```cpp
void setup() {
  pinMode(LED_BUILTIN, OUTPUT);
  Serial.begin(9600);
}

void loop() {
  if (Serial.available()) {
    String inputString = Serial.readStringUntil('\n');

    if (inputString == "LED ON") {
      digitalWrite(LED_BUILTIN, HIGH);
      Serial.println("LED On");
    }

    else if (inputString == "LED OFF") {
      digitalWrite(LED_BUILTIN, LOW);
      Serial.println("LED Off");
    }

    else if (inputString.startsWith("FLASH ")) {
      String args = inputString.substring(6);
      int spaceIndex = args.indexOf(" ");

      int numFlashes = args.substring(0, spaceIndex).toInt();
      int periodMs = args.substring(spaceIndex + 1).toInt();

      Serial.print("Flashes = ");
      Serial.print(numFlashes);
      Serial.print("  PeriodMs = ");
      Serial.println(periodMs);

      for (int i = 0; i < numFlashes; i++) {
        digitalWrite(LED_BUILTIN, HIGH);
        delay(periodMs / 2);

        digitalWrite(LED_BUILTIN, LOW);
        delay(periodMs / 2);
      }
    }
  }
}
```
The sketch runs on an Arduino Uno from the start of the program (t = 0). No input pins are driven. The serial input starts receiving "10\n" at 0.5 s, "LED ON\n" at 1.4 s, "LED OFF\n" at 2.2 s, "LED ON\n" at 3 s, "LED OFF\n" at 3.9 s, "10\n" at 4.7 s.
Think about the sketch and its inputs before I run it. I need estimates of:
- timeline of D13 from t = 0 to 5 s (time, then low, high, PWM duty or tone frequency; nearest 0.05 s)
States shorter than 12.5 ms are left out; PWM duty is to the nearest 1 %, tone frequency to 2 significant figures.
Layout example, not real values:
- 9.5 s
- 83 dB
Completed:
- 0 s low; 1.4 s high; 2.2 s low; 3 s high; 3.9 s low
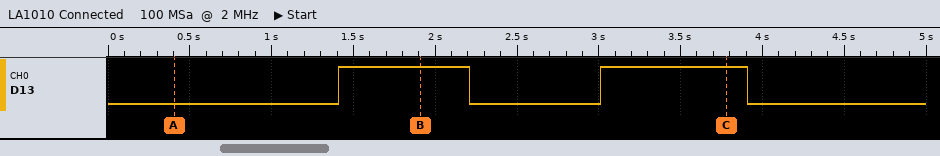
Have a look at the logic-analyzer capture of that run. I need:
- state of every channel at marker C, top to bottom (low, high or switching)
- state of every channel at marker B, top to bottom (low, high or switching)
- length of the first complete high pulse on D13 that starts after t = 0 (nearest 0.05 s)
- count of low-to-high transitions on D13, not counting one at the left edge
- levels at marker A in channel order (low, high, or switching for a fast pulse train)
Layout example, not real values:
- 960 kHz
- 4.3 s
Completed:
- D13 high
- D13 high
- 0.80 s
- 2
- D13 low
